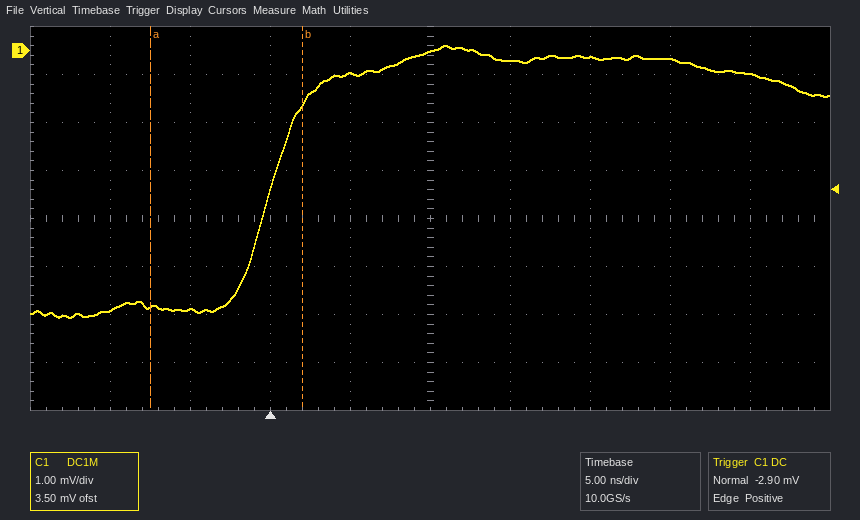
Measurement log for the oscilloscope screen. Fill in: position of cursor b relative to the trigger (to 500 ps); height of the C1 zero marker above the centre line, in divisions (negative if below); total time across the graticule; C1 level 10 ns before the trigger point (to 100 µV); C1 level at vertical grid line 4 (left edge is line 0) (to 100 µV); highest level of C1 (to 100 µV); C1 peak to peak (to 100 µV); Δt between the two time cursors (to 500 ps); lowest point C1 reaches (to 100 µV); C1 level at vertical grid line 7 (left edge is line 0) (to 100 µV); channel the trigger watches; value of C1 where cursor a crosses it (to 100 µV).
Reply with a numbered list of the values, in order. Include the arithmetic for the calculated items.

1. +2.0 ns
2. +3.5 div
3. 50 ns
4. -5.4 mV
5. -500 µV
6. 100 µV
7. 100 µV − (-5.6 mV) = 5.7 mV
8. 9.5 ns
9. -5.6 mV
10. -100 µV
11. C1
12. -5.3 mV
